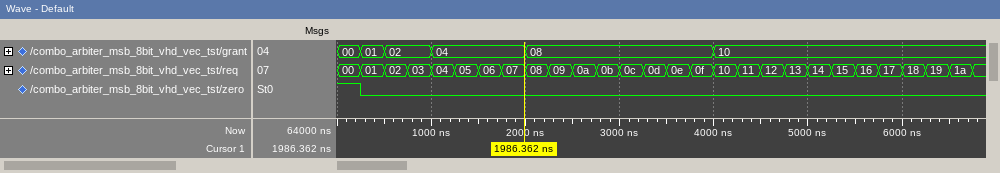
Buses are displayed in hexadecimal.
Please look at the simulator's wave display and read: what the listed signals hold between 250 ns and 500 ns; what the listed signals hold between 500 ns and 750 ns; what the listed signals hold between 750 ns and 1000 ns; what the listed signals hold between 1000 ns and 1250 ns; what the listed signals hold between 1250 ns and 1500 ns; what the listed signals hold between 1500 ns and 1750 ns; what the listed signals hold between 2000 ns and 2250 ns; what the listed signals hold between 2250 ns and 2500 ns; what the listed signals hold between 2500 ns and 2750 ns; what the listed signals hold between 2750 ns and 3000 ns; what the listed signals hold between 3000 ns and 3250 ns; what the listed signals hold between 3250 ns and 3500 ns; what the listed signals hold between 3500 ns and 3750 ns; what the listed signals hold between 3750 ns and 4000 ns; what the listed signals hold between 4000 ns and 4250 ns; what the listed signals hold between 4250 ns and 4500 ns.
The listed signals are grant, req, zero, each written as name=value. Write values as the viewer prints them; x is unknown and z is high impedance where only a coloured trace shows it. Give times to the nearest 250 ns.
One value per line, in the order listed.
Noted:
grant=01, req=01, zero=0
grant=02, req=02, zero=0
grant=02, req=03, zero=0
grant=04, req=04, zero=0
grant=04, req=05, zero=0
grant=04, req=06, zero=0
grant=08, req=08, zero=0
grant=08, req=09, zero=0
grant=08, req=0a, zero=0
grant=08, req=0b, zero=0
grant=08, req=0c, zero=0
grant=08, req=0d, zero=0
grant=08, req=0e, zero=0
grant=08, req=0f, zero=0
grant=10, req=10, zero=0
grant=10, req=11, zero=0
